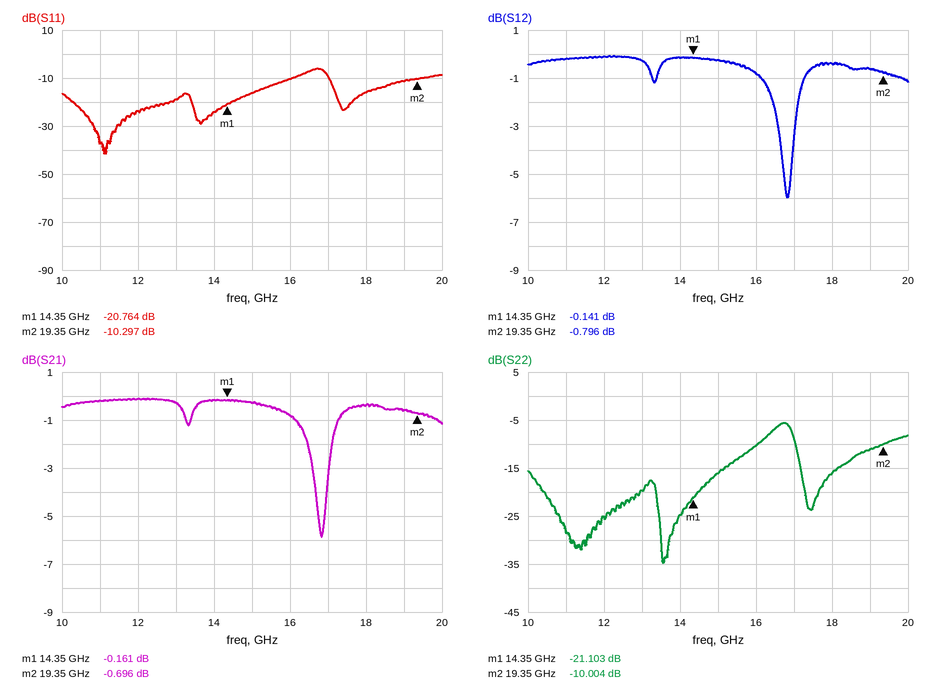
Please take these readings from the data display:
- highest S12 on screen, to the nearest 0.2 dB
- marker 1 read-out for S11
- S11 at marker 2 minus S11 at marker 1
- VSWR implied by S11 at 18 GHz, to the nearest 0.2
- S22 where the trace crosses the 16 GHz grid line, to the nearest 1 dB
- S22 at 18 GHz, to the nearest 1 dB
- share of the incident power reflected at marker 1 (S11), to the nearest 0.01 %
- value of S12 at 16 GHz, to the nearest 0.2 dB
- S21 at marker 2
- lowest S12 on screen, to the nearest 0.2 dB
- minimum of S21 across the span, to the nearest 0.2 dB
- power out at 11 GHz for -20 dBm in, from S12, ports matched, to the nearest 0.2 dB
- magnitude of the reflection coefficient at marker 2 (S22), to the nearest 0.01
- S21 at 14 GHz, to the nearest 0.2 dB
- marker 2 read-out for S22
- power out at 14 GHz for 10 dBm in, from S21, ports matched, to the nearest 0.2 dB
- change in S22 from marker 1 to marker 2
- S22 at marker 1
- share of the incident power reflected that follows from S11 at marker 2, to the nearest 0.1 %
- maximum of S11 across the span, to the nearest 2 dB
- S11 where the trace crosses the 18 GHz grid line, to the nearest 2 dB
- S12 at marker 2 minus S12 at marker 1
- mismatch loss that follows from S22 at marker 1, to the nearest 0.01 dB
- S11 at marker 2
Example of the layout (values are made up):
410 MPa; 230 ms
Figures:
0.0 dB; -20.764 dB; 10.467 dB; 1.4; -10 dB; -16 dB; 0.84 %; -0.8 dB; -0.696 dB; -6.0 dB; -5.8 dB; -20.2 dBm; 0.32; -0.2 dB; -10.004 dB; 9.8 dBm; 11.099 dB; -21.103 dB; 9.3 %; -6 dB; -16 dB; -0.655 dB; 0.03 dB; -10.297 dB
